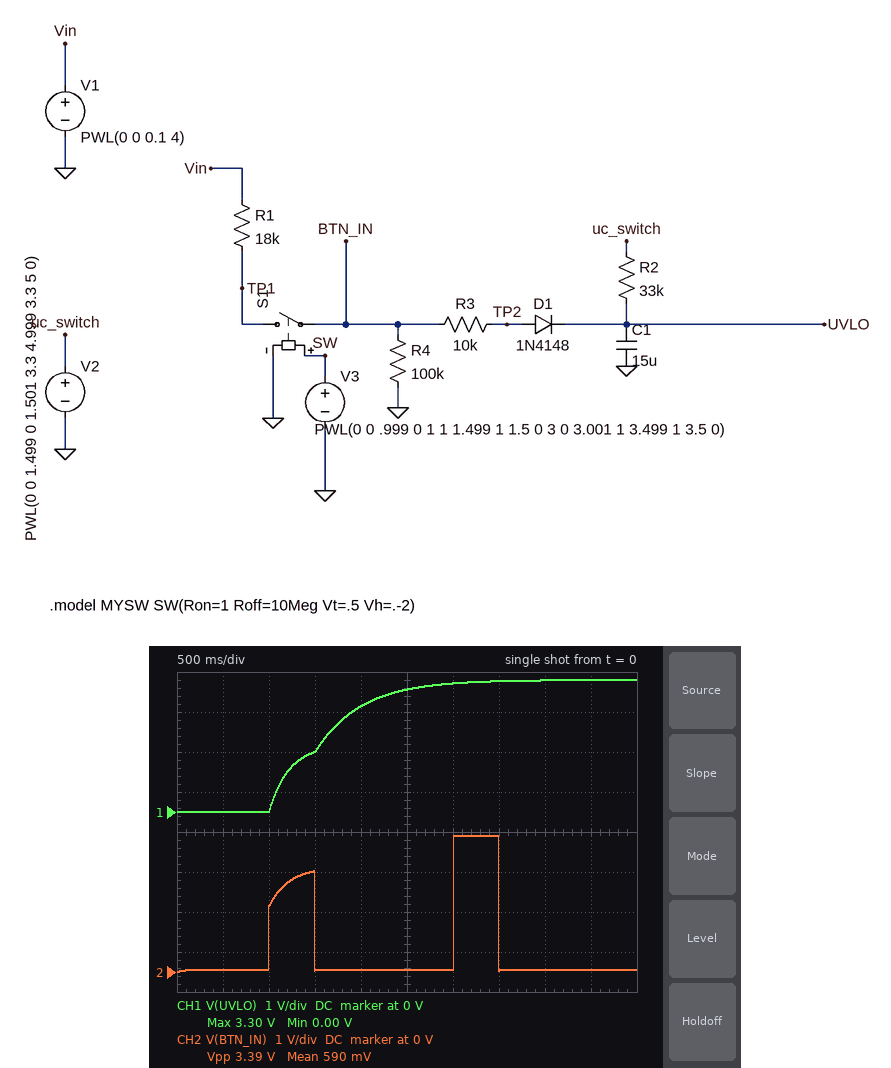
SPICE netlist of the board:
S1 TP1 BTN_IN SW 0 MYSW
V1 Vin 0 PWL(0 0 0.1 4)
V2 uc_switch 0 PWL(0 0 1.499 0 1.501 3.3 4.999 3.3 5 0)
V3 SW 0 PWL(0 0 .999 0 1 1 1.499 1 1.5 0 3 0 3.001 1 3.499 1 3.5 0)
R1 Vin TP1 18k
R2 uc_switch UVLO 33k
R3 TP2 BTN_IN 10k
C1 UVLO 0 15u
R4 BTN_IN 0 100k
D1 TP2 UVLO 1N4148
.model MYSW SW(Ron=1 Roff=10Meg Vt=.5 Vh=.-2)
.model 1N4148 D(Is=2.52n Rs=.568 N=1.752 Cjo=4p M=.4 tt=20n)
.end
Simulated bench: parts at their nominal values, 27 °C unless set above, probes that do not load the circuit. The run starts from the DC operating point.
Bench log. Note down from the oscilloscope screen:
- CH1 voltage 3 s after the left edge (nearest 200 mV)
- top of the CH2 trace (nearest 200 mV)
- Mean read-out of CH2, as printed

3.2 V
3.4 V
590 mV
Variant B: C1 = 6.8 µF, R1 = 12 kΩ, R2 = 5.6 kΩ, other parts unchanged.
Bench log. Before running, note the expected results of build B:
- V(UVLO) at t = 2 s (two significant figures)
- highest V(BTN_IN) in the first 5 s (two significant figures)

3.3 V
3.6 V
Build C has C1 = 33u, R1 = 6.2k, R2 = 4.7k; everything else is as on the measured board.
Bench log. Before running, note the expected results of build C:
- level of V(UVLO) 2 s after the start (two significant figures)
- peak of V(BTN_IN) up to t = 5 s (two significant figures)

3.2 V
3.7 V
